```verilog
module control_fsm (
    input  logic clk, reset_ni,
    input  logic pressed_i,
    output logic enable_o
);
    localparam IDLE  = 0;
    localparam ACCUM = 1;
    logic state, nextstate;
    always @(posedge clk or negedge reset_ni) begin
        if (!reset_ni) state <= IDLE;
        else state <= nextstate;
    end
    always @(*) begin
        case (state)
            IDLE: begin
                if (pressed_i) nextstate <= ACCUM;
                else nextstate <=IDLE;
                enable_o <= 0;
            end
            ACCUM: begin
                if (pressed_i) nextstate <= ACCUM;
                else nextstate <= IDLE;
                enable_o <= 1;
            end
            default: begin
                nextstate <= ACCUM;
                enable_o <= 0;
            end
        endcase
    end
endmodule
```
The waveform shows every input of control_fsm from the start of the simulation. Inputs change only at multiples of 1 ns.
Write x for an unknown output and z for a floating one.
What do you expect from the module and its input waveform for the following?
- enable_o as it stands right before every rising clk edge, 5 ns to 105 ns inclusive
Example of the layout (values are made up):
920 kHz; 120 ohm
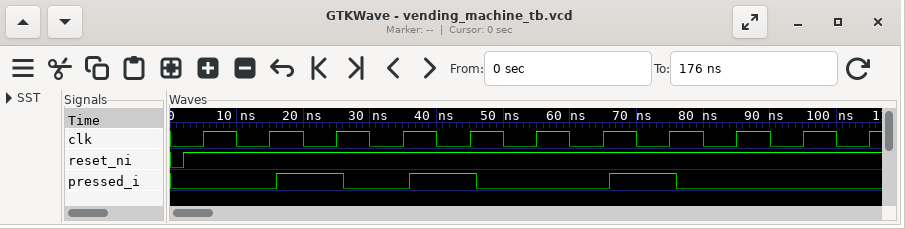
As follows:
0 0 0 1 0 1 0 0 1 0 0
